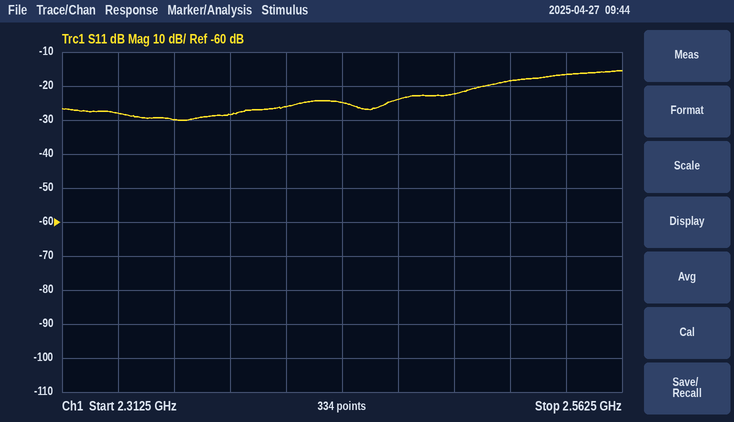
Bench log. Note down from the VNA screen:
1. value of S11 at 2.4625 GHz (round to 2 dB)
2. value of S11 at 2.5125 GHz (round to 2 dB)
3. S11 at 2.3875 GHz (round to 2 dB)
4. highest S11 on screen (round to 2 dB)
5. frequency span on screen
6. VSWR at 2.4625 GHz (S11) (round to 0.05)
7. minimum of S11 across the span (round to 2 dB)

-24 dB
-18 dB
-28 dB
-16 dB
250 MHz
1.15
-30 dB
